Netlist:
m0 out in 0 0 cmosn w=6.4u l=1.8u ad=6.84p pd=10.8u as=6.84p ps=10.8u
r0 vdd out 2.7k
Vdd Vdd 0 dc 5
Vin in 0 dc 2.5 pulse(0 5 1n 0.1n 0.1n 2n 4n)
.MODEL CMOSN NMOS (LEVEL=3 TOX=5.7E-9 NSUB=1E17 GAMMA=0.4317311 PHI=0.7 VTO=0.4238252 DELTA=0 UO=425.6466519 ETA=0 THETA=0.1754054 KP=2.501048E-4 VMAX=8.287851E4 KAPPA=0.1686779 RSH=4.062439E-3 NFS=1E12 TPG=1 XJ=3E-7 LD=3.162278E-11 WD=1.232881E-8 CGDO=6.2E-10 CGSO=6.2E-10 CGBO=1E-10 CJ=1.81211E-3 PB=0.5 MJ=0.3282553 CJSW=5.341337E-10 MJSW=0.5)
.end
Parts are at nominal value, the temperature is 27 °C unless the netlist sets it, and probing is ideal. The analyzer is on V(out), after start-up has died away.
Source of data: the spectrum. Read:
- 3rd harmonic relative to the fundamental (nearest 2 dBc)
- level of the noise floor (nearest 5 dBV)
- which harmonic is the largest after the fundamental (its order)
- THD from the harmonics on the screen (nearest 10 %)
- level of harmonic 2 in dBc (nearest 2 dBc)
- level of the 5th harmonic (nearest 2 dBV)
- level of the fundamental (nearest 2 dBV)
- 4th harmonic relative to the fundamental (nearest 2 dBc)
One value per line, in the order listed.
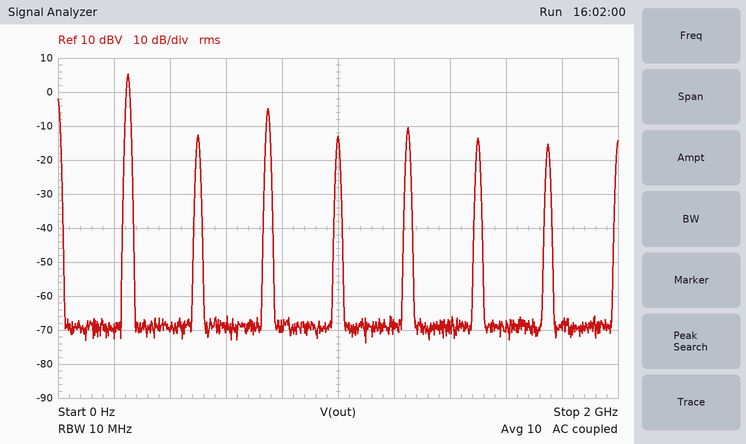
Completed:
-10 dBc
-70 dBV
3
40 %
-18 dBc
-10 dBV
6 dBV
-18 dBc
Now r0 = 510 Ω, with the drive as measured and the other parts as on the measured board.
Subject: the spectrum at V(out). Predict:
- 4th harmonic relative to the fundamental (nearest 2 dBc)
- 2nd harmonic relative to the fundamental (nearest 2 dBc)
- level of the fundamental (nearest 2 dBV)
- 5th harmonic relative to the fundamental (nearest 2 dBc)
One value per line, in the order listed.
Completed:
-24 dBc
-24 dBc
-4 dBV
-14 dBc
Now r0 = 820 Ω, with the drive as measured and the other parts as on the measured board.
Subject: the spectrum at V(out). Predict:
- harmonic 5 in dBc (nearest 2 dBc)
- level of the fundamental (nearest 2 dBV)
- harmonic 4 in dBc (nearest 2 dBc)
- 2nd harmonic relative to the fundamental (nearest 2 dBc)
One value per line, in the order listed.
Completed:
-14 dBc
0 dBV
-24 dBc
-24 dBc
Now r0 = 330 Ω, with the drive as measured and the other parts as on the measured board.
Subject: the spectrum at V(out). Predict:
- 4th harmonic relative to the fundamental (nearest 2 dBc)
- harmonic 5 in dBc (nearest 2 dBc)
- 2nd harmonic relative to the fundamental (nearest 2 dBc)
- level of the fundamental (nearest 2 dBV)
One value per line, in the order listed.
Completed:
-24 dBc
-14 dBc
-24 dBc
-8 dBV
